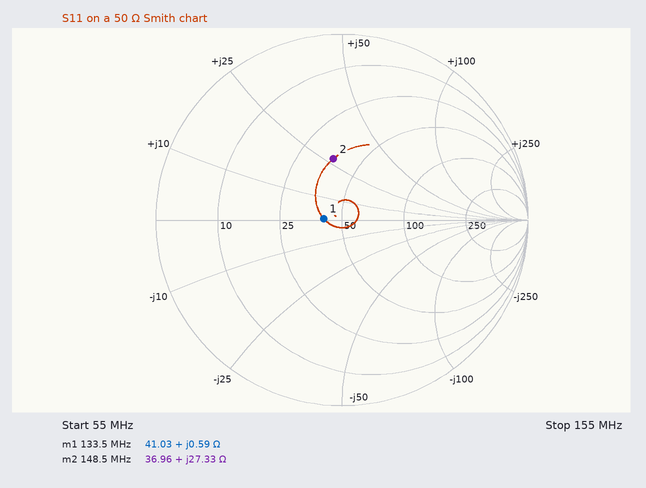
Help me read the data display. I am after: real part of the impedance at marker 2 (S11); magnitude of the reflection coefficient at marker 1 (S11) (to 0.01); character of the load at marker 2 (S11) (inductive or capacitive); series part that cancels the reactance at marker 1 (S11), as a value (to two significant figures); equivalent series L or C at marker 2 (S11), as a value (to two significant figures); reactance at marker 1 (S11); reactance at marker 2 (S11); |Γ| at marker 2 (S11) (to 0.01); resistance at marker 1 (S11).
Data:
36.96 Ω
0.10
inductive
2.0 nF
29 nH
+0.59 Ω
+27.33 Ω
0.33
41.03 Ω
